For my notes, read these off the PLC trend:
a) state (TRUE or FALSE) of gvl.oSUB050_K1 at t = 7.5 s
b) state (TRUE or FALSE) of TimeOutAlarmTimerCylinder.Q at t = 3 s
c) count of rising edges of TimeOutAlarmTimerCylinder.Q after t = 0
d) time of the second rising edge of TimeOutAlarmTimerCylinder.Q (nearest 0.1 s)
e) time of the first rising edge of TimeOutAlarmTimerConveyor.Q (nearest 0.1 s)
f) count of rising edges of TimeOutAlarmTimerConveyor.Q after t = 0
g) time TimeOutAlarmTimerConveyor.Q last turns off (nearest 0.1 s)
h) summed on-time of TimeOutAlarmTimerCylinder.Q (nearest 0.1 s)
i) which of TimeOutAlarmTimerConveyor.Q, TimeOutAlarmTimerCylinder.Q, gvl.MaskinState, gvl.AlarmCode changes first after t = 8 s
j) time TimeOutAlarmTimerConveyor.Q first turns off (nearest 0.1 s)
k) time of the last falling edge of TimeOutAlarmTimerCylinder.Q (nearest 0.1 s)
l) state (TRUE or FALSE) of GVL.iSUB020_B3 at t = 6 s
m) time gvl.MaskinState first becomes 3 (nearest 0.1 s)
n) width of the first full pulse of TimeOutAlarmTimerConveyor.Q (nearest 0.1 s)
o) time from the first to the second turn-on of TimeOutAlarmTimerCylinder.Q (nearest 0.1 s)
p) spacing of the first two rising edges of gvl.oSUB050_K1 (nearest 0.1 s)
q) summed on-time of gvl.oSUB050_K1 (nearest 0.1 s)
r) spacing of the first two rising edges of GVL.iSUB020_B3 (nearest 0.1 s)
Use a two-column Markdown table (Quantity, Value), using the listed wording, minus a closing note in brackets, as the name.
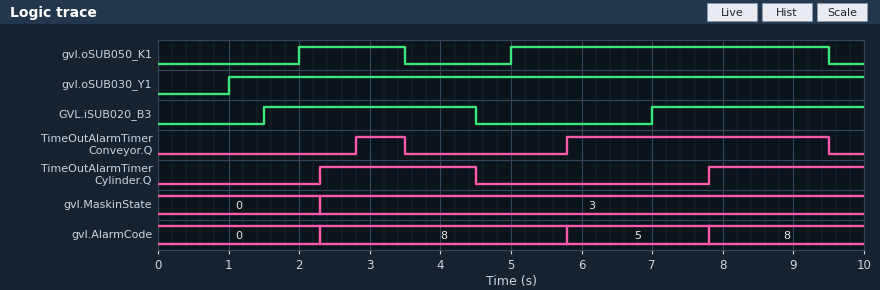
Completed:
| Quantity | Value |
|---|---|
| state (TRUE or FALSE) of gvl.oSUB050_K1 at t = 7.5 s | TRUE |
| state (TRUE or FALSE) of TimeOutAlarmTimerCylinder.Q at t = 3 s | TRUE |
| count of rising edges of TimeOutAlarmTimerCylinder.Q after t = 0 | 2 |
| time of the second rising edge of TimeOutAlarmTimerCylinder.Q | 7.8 s |
| time of the first rising edge of TimeOutAlarmTimerConveyor.Q | 2.8 s |
| count of rising edges of TimeOutAlarmTimerConveyor.Q after t = 0 | 2 |
| time TimeOutAlarmTimerConveyor.Q last turns off | 9.5 s |
| summed on-time of TimeOutAlarmTimerCylinder.Q | 4.4 s |
| which of TimeOutAlarmTimerConveyor.Q, TimeOutAlarmTimerCylinder.Q, gvl.MaskinState, gvl.AlarmCode changes first after t = 8 s | TimeOutAlarmTimerConveyor.Q |
| time TimeOutAlarmTimerConveyor.Q first turns off | 3.5 s |
| time of the last falling edge of TimeOutAlarmTimerCylinder.Q | 4.5 s |
| state (TRUE or FALSE) of GVL.iSUB020_B3 at t = 6 s | FALSE |
| time gvl.MaskinState first becomes 3 | 2.3 s |
| width of the first full pulse of TimeOutAlarmTimerConveyor.Q | 0.7 s |
| time from the first to the second turn-on of TimeOutAlarmTimerCylinder.Q | 5.5 s |
| spacing of the first two rising edges of gvl.oSUB050_K1 | 3.0 s |
| summed on-time of gvl.oSUB050_K1 | 6.0 s |
| spacing of the first two rising edges of GVL.iSUB020_B3 | 5.5 s |
